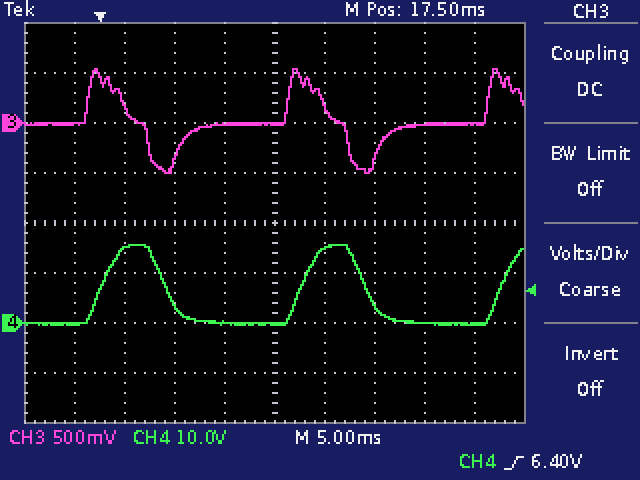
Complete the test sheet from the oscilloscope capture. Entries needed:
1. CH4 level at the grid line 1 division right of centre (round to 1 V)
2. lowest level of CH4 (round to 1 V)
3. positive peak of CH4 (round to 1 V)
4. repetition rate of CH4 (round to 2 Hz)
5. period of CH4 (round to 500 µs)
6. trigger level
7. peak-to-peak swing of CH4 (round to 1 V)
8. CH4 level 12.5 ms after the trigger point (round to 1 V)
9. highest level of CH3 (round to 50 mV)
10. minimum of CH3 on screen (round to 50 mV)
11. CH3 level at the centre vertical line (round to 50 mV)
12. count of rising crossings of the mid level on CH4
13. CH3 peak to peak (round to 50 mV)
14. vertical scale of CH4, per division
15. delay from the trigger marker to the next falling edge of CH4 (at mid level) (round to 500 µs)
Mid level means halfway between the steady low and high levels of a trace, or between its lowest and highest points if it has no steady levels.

15 V
0 V
16 V
50 Hz
20.0 ms
6.40 V
16 V
0 V
550 mV
-500 mV
0 mV
3
1.05 V
10 V
6.5 ms
